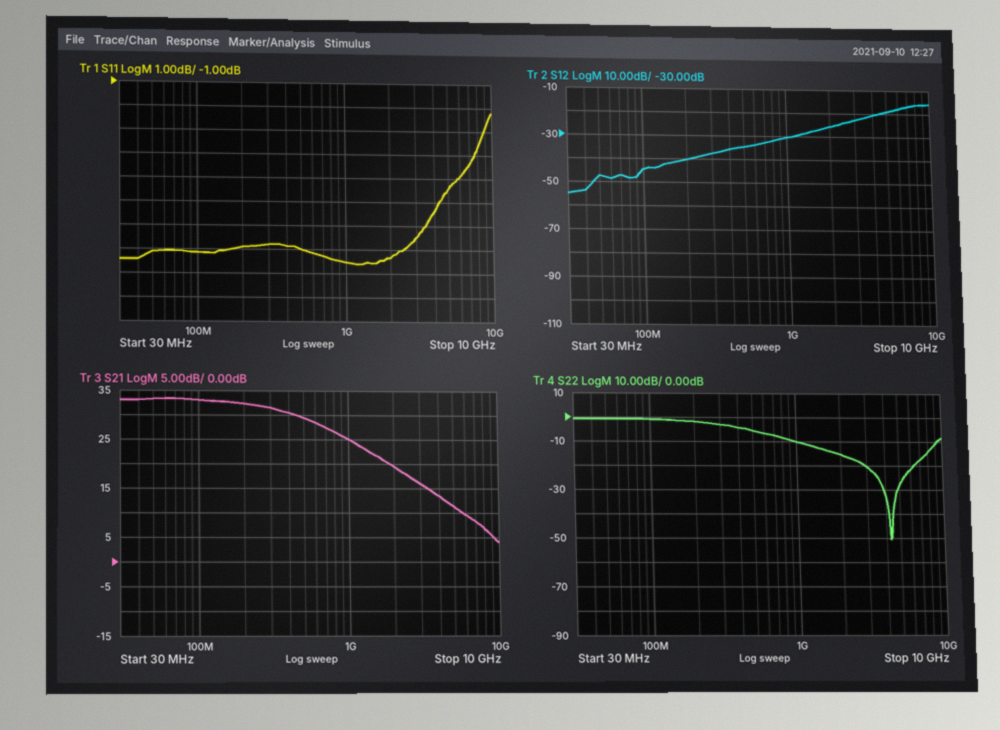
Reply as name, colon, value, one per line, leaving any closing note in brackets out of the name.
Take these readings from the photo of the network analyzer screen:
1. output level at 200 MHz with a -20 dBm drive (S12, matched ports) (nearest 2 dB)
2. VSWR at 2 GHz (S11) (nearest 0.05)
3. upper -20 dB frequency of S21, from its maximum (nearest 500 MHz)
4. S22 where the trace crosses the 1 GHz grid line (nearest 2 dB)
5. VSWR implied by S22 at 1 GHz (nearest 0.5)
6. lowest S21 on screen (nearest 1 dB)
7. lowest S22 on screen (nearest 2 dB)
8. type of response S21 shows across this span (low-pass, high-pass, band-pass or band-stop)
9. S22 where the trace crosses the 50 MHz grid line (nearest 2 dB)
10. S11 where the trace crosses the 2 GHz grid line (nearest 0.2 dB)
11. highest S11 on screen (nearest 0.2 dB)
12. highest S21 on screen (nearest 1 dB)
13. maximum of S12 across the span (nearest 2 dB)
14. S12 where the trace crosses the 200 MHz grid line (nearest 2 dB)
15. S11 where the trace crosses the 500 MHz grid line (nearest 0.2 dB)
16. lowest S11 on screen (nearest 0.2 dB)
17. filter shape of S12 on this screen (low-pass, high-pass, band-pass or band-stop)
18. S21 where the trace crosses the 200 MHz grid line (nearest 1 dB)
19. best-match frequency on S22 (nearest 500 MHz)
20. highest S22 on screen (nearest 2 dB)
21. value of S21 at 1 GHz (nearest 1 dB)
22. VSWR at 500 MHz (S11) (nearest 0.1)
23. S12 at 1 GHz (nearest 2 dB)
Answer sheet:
output level at 200 MHz with a -20 dBm drive (S12, matched ports): -60 dBm
VSWR at 2 GHz (S11): 2.25
upper -20 dB frequency of S21, from its maximum: 4.0 GHz
S22 where the trace crosses the 1 GHz grid line: -10 dB
VSWR implied by S22 at 1 GHz: 2.0
lowest S21 on screen: 4 dB
lowest S22 on screen: -50 dB
type of response S21 shows across this span: low-pass
S22 where the trace crosses the 50 MHz grid line: 0 dB
S11 where the trace crosses the 2 GHz grid line: -8.4 dB
highest S11 on screen: -2.2 dB
highest S21 on screen: 33 dB
maximum of S12 across the span: -16 dB
S12 where the trace crosses the 200 MHz grid line: -40 dB
S11 where the trace crosses the 500 MHz grid line: -8.0 dB
lowest S11 on screen: -8.6 dB
filter shape of S12 on this screen: high-pass
S21 where the trace crosses the 200 MHz grid line: 32 dB
best-match frequency on S22: 4.5 GHz
highest S22 on screen: 0 dB
value of S21 at 1 GHz: 25 dB
VSWR at 500 MHz (S11): 2.3
S12 at 1 GHz: -30 dB
